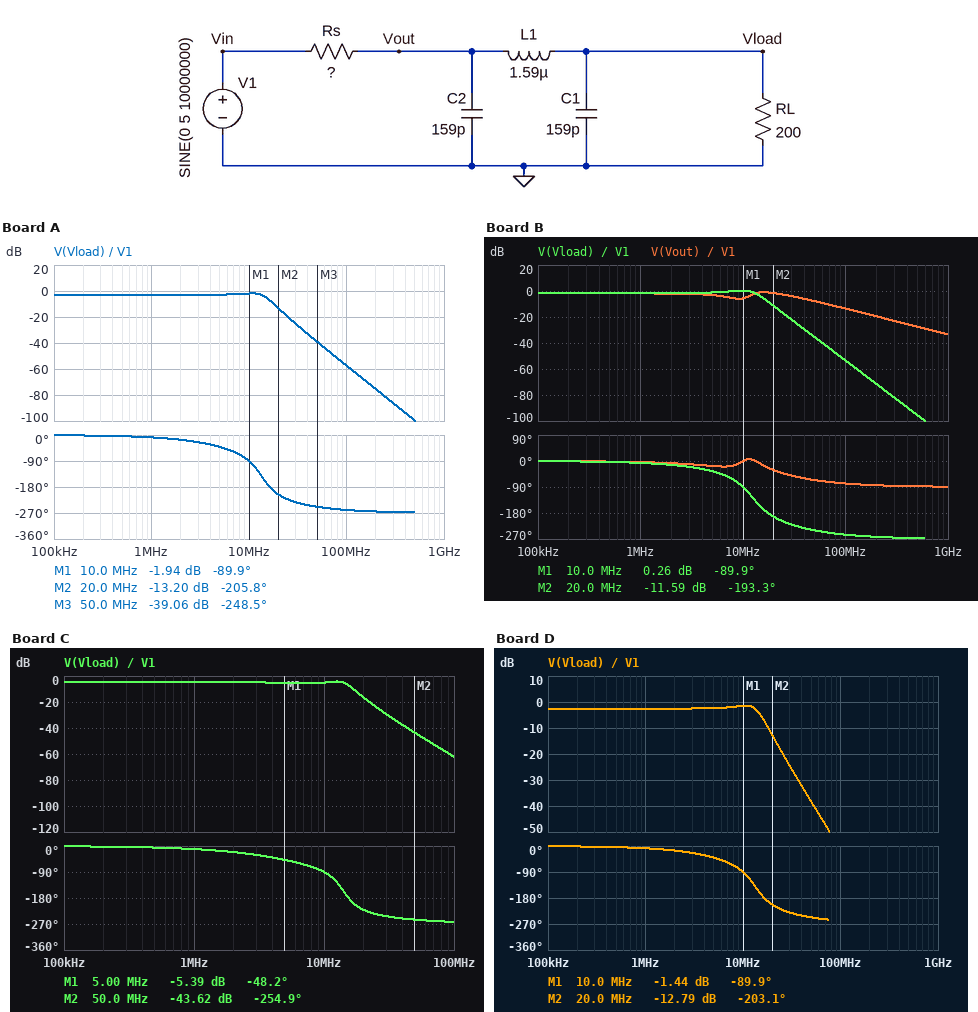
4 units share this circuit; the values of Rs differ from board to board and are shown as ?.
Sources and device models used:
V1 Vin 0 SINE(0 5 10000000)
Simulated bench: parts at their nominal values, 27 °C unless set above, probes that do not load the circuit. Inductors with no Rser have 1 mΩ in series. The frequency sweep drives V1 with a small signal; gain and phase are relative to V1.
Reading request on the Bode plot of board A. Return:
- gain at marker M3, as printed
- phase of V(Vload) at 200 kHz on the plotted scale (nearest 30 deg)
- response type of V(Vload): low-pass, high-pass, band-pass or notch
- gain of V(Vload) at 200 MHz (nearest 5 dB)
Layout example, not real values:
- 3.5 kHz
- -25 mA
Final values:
- -39.06 dB
- 0 deg
- low-pass
- -75 dB
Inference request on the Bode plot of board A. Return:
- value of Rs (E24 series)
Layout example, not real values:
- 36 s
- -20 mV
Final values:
- 75 Ω
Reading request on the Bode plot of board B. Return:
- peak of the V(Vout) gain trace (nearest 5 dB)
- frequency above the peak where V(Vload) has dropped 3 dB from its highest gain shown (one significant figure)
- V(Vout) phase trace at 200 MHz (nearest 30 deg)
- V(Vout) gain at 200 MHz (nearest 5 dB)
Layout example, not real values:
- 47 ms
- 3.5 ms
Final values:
- 0 dB
- 10 MHz
- -90 deg
- -20 dB
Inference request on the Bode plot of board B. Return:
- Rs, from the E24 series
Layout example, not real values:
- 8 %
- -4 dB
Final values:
- 47 Ω
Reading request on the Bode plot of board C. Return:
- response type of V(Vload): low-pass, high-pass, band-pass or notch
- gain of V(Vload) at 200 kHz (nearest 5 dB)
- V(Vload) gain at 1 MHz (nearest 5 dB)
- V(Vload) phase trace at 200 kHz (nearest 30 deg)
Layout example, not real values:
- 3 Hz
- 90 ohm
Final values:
- low-pass
- -5 dB
- -5 dB
- 0 deg
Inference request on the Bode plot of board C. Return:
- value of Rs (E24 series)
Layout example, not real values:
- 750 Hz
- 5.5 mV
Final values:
- 130 Ω
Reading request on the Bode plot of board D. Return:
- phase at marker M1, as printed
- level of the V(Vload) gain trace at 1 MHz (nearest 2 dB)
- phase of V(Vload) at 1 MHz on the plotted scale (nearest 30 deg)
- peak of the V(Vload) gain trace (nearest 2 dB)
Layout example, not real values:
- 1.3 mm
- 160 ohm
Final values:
- -89.9 deg
- -2 dB
- 0 deg
- -2 dB
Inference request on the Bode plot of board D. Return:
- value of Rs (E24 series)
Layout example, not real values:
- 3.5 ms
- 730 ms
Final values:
- 68 Ω
